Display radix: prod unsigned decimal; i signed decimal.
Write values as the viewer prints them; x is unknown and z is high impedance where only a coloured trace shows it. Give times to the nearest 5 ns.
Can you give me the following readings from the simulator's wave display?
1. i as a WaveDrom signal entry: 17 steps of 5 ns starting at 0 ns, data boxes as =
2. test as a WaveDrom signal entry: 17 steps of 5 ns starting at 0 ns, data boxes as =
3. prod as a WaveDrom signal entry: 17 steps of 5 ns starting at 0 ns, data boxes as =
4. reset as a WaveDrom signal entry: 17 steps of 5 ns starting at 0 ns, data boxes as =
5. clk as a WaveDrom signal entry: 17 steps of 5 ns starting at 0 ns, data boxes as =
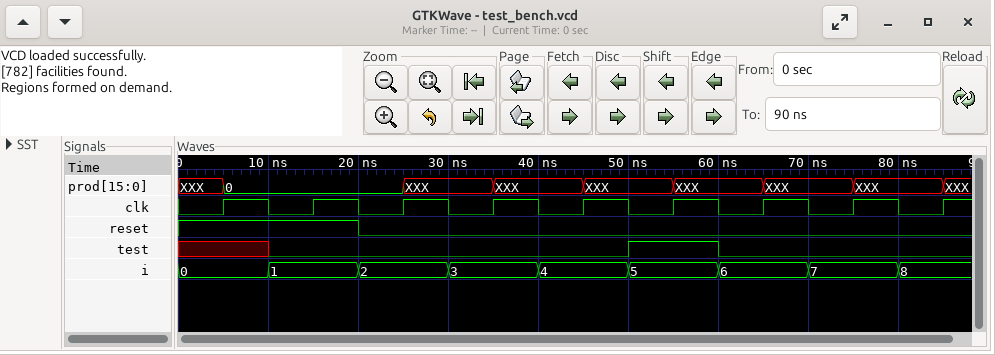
{name: 'i', wave: '=.=.=.=.=.=.=.=.=', data: '0 1 2 3 4 5 6 7 8'}
{name: 'test', wave: 'x.0.......1.0....'}
{name: 'prod', wave: 'x=...=.=.=.=.=.=.', data: '0 XXX XXX XXX XXX XXX XXX'}
{name: 'reset', wave: '1...0............'}
{name: 'clk', wave: '01010101010101010'}
